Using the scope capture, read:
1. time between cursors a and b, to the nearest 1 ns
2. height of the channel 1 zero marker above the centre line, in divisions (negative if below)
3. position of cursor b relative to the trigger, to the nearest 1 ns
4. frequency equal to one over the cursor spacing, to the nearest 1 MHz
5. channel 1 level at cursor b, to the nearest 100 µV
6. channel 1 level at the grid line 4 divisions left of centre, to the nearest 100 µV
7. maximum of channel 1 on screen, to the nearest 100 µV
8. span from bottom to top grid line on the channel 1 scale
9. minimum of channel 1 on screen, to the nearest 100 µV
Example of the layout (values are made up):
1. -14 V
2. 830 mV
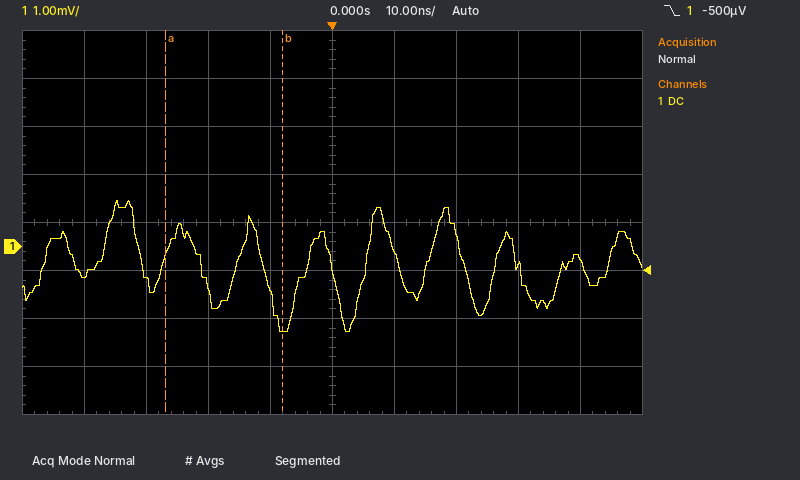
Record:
1. 19 ns
2. -0.5 div
3. -8 ns
4. 53 MHz
5. -1.7 mV
6. -600 µV
7. 1.0 mV
8. 8 mV
9. -1.8 mV
